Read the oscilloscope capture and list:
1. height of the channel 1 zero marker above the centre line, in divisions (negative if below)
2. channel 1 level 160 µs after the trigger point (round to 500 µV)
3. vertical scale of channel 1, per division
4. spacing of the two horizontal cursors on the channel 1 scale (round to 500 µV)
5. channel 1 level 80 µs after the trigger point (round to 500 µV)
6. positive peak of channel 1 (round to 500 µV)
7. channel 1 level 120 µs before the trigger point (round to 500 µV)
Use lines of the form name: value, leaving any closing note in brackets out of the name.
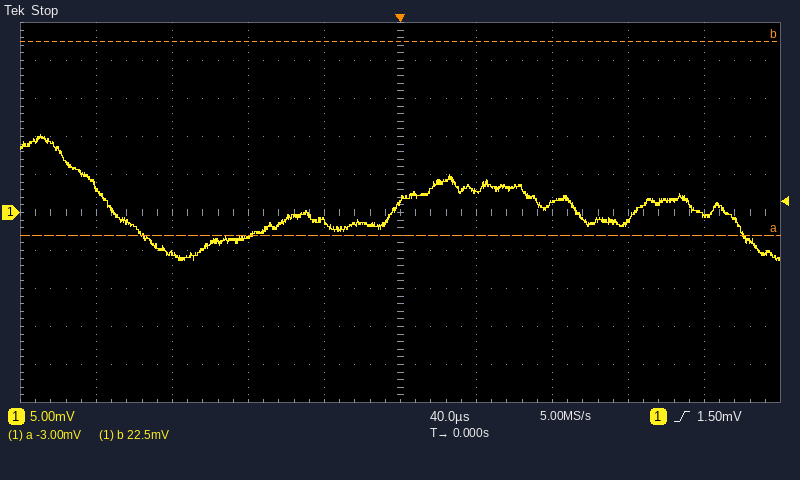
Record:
height of the channel 1 zero marker above the centre line, in divisions: 0.0 div
channel 1 level 160 µs after the trigger point: -500 µV
vertical scale of channel 1, per division: 5 mV
spacing of the two horizontal cursors on the channel 1 scale: 25.5 mV
channel 1 level 80 µs after the trigger point: 1.0 mV
positive peak of channel 1: 10.5 mV
channel 1 level 120 µs before the trigger point: -5.5 mV
